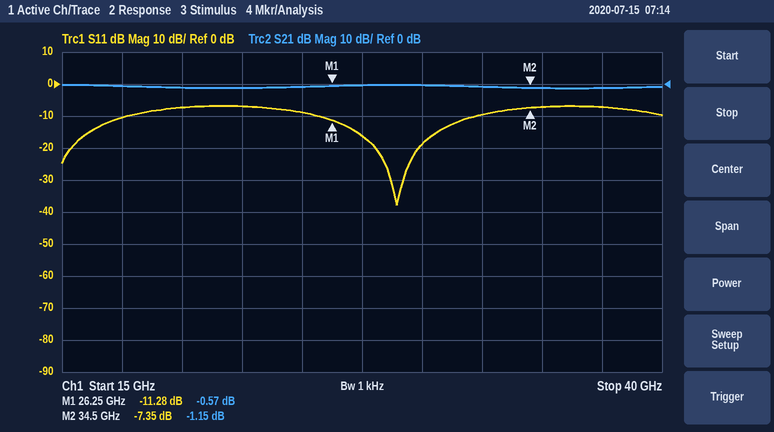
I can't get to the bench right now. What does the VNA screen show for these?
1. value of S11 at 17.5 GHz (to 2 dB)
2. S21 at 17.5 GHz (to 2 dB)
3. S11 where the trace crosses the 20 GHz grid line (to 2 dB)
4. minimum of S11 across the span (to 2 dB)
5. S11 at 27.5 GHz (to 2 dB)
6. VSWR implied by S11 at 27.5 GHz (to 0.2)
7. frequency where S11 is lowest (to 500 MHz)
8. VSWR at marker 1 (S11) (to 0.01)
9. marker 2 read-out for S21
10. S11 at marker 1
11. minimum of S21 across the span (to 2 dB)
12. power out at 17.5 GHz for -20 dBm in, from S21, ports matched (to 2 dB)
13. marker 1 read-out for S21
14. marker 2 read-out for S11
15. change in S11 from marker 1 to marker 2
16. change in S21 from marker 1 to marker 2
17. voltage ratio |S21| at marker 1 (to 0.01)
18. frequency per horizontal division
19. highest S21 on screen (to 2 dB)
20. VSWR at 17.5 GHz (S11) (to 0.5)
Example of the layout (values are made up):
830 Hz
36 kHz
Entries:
-10 dB
0 dB
-8 dB
-38 dB
-16 dB
1.4
29.0 GHz
1.75
-1.15 dB
-11.28 dB
-2 dB
-20 dBm
-0.57 dB
-7.35 dB
3.93 dB
-0.58 dB
0.94
2.5 GHz
0 dB
2.0
